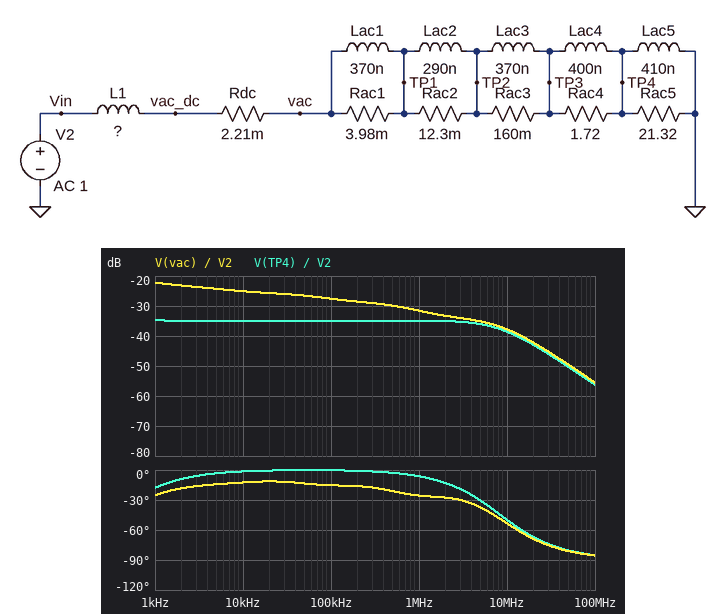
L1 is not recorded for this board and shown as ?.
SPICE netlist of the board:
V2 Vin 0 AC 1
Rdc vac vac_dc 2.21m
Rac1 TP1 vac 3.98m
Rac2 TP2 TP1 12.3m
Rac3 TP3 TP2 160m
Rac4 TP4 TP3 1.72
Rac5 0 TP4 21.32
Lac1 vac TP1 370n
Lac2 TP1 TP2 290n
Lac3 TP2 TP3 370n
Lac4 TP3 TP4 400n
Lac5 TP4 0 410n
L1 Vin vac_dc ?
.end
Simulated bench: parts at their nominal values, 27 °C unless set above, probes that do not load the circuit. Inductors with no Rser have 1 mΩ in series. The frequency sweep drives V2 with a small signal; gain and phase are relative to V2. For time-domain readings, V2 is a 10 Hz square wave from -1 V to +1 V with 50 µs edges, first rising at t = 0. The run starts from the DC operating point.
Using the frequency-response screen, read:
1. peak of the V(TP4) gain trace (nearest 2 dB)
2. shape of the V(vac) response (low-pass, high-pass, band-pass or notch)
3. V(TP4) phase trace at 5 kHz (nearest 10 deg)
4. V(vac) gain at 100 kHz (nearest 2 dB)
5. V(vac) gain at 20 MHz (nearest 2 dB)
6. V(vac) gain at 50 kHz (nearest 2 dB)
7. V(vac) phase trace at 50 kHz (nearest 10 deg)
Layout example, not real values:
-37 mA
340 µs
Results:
-34 dB
low-pass
0 deg
-28 dB
-42 dB
-26 dB
-10 deg
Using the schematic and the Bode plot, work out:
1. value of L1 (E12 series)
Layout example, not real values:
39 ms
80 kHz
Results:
22 µH
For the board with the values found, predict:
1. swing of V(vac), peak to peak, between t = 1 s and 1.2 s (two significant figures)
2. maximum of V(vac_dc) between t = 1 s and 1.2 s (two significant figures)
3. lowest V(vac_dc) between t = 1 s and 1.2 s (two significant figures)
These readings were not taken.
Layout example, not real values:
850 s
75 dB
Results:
1.2 V
870 mV
-870 mV
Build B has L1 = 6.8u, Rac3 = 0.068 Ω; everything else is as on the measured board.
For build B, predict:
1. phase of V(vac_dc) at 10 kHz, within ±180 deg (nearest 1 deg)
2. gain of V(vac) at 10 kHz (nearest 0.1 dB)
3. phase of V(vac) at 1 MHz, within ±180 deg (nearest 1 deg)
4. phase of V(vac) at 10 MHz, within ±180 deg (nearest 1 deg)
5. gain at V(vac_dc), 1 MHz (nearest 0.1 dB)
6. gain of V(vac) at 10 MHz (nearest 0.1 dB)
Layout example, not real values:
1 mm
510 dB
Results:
-15 deg
-16.0 dB
-23 deg
-52 deg
-21.9 dB
-27.8 dB
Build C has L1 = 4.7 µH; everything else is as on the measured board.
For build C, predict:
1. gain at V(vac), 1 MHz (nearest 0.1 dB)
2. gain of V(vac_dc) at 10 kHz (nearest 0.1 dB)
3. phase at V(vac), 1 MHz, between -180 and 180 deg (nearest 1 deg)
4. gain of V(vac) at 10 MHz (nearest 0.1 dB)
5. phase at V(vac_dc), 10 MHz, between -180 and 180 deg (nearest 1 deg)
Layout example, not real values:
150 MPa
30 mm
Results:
-18.9 dB
-13.2 dB
-23 deg
-24.6 dB
-51 deg
